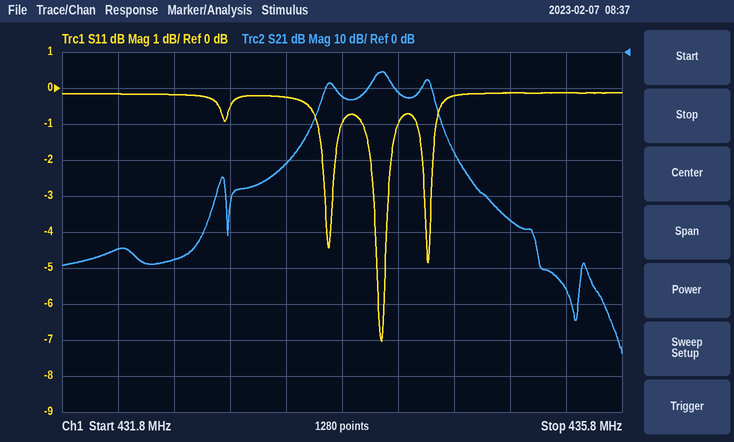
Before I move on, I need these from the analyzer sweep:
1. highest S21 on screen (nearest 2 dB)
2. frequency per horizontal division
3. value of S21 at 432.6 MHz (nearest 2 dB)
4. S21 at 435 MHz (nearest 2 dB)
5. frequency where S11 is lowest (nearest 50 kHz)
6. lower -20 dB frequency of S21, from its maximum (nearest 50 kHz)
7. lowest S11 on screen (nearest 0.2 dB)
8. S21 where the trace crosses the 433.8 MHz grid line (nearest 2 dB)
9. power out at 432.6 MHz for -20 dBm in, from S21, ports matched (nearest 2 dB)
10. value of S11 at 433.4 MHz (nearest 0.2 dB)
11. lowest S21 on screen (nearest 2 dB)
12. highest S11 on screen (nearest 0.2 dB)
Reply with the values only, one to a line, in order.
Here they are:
-6 dB
400 kHz
-58 dB
-46 dB
434.10 MHz
433.50 MHz
-7.0 dB
-12 dB
-78 dBm
-0.2 dB
-84 dB
-0.2 dB
